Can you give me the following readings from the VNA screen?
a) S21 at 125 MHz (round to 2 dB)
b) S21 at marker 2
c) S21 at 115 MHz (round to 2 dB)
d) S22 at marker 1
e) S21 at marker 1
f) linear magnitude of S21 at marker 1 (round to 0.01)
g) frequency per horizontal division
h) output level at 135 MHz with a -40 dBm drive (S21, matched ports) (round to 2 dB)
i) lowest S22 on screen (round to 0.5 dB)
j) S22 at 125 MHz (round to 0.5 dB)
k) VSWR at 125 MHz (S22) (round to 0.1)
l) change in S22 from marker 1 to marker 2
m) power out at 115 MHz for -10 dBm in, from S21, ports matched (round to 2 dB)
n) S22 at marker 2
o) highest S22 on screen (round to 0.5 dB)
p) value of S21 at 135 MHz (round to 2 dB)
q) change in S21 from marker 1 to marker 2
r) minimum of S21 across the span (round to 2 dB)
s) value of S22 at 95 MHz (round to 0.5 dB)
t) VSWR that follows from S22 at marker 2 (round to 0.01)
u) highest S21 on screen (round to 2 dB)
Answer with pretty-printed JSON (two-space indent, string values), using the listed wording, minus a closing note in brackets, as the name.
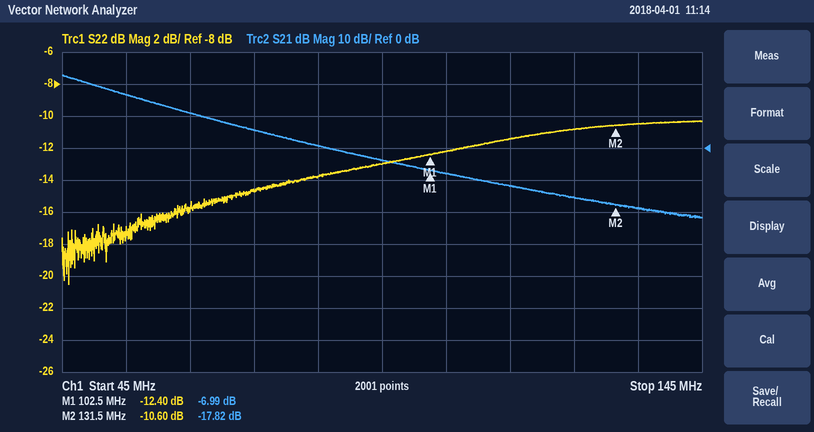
{
  "S21 at 125 MHz": "-16 dB",
  "S21 at marker 2": "-17.82 dB",
  "S21 at 115 MHz": "-12 dB",
  "S22 at marker 1": "-12.40 dB",
  "S21 at marker 1": "-6.99 dB",
  "linear magnitude of S21 at marker 1": "0.45",
  "frequency per horizontal division": "10 MHz",
  "output level at 135 MHz with a -40 dBm drive (S21, matched ports)": "-58 dBm",
  "lowest S22 on screen": "-20.5 dB",
  "S22 at 125 MHz": "-11.0 dB",
  "VSWR at 125 MHz (S22)": "1.8",
  "change in S22 from marker 1 to marker 2": "1.80 dB",
  "power out at 115 MHz for -10 dBm in, from S21, ports matched": "-22 dBm",
  "S22 at marker 2": "-10.60 dB",
  "highest S22 on screen": "-10.5 dB",
  "value of S21 at 135 MHz": "-18 dB",
  "change in S21 from marker 1 to marker 2": "-10.83 dB",
  "minimum of S21 across the span": "-22 dB",
  "value of S22 at 95 MHz": "-13.0 dB",
  "VSWR that follows from S22 at marker 2": "1.84",
  "highest S21 on screen": "22 dB"
}
